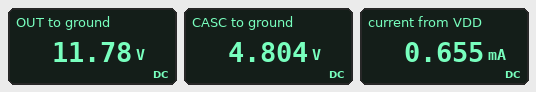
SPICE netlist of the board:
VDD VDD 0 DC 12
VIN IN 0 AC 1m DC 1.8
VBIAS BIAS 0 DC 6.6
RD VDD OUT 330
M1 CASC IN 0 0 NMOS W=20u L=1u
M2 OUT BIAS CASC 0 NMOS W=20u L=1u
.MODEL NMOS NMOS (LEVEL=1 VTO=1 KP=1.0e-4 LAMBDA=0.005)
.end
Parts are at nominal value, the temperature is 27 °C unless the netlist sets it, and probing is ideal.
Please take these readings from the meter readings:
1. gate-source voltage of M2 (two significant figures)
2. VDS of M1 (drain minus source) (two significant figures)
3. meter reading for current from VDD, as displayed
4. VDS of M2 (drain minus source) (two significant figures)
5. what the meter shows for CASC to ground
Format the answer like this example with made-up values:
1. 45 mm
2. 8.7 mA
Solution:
1. 1.8 V
2. 4.8 V
3. 0.655 mA
4. 7.0 V
5. 4.804 V
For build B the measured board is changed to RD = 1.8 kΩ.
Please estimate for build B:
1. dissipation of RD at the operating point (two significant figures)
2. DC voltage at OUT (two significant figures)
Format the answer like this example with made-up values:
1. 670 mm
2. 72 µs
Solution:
1. 770 µW
2. 11 V
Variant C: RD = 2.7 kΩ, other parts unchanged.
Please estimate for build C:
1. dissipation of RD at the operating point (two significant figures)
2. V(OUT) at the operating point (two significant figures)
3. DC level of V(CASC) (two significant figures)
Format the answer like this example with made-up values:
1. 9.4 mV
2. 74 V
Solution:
1. 1.2 mW
2. 10 V
3. 4.8 V
